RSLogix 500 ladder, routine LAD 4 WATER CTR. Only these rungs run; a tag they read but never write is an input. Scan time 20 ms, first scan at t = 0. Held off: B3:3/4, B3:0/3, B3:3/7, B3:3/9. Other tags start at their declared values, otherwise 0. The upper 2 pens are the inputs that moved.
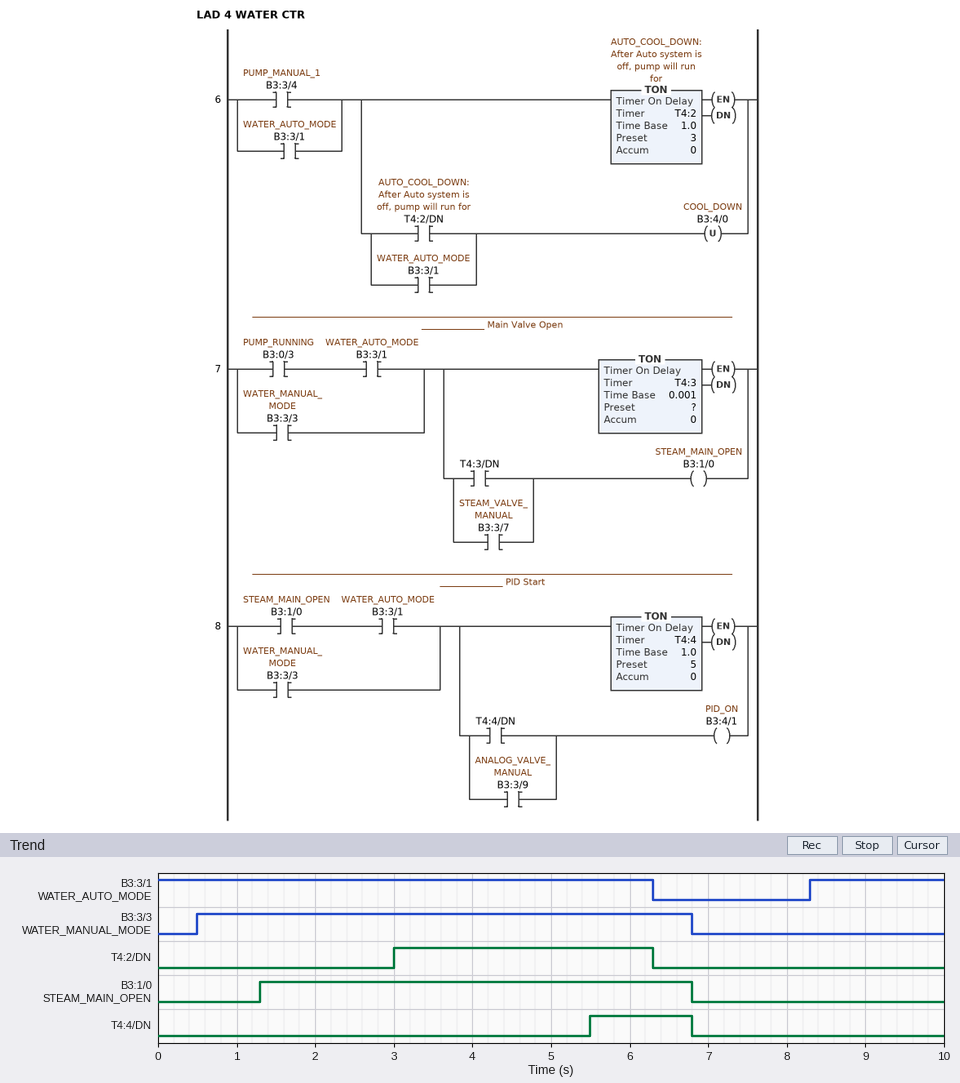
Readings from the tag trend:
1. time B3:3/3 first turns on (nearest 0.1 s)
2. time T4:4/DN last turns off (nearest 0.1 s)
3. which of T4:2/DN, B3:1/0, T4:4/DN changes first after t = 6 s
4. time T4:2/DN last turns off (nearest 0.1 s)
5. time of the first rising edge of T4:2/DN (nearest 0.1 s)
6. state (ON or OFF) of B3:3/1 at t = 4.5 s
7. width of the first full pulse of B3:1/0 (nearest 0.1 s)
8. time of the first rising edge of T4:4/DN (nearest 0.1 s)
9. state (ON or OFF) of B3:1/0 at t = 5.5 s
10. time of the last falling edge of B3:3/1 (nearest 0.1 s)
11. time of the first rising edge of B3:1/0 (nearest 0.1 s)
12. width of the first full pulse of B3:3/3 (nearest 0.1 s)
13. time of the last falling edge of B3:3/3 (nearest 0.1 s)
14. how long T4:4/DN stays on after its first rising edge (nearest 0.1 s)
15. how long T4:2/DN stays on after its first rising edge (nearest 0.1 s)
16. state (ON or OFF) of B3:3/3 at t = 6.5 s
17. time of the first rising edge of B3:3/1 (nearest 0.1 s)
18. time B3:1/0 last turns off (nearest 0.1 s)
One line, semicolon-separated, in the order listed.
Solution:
0.5 s; 6.8 s; T4:2/DN; 6.3 s; 3.0 s; ON; 5.5 s; 5.5 s; ON; 6.3 s; 1.3 s; 6.3 s; 6.8 s; 1.3 s; 3.3 s; ON; 8.3 s; 6.8 s
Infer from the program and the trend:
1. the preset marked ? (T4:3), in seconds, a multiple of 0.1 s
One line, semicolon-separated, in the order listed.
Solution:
0.8 s
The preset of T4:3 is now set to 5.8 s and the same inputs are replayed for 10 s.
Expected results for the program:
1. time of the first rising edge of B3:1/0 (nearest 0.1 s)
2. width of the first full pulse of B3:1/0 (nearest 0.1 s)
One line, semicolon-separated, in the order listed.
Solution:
6.3 s; 0.5 s
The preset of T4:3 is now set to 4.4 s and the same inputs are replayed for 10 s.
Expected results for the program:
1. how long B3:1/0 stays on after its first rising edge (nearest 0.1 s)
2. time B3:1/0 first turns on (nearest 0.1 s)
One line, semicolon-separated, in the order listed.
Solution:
1.9 s; 4.9 s
